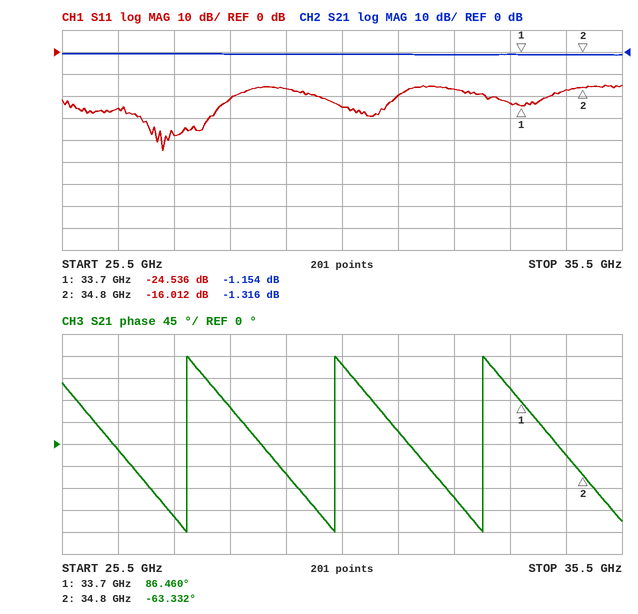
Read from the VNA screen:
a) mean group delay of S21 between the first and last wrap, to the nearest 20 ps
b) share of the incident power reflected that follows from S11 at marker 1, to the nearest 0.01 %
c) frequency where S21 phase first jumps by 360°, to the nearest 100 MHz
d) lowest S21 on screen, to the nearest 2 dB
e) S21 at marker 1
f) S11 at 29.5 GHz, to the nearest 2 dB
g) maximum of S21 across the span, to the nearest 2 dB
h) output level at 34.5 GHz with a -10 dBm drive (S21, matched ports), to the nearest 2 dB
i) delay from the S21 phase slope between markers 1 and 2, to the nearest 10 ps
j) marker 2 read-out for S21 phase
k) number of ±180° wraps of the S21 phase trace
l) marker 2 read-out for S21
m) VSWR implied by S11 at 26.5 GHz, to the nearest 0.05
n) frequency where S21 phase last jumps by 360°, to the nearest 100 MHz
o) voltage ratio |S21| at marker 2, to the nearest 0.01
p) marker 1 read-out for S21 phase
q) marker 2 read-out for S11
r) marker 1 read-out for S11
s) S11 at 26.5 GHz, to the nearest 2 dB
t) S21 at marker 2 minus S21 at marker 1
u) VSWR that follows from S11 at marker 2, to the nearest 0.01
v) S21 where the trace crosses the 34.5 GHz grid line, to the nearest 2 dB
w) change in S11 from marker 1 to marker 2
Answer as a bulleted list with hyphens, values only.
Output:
- 380 ps
- 0.35 %
- 27.7 GHz
- -2 dB
- -1.154 dB
- -16 dB
- 0 dB
- -12 dBm
- 380 ps
- -63.332°
- 3
- -1.316 dB
- 1.10
- 33.0 GHz
- 0.86
- 86.460°
- -16.012 dB
- -24.536 dB
- -26 dB
- -0.162 dB
- 1.38
- -2 dB
- 8.524 dB
